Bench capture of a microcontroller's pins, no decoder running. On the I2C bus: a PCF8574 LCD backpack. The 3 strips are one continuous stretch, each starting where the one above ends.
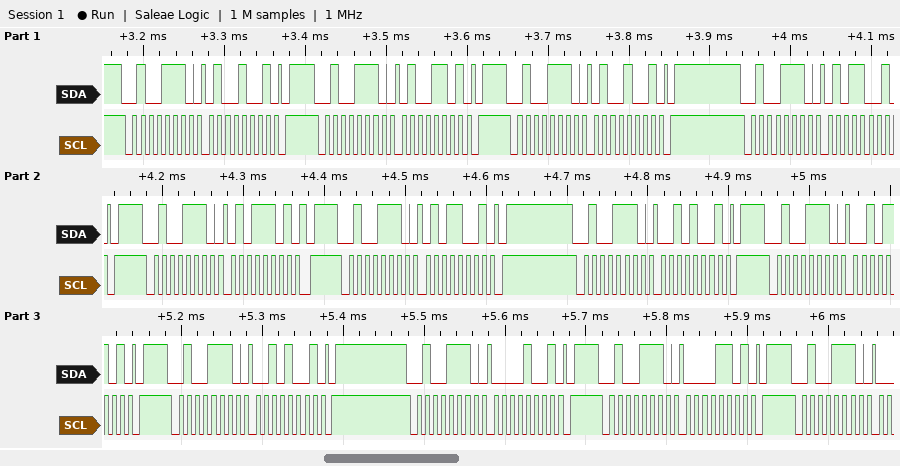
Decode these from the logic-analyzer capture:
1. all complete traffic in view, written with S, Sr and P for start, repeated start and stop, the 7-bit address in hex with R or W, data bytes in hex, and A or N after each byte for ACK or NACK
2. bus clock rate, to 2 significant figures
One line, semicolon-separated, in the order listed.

S 27W A 49 A P S 27W A 4D A P S 27W A 49 A P S 27W A 59 A P S 27W A 5D A P S 27W A 59 A P S 27W A 29 A P S 27W A 2D A P S 27W A 29 A P S 27W A 09 A P S 27W A 0D A P S 27W A; 100 kHz
